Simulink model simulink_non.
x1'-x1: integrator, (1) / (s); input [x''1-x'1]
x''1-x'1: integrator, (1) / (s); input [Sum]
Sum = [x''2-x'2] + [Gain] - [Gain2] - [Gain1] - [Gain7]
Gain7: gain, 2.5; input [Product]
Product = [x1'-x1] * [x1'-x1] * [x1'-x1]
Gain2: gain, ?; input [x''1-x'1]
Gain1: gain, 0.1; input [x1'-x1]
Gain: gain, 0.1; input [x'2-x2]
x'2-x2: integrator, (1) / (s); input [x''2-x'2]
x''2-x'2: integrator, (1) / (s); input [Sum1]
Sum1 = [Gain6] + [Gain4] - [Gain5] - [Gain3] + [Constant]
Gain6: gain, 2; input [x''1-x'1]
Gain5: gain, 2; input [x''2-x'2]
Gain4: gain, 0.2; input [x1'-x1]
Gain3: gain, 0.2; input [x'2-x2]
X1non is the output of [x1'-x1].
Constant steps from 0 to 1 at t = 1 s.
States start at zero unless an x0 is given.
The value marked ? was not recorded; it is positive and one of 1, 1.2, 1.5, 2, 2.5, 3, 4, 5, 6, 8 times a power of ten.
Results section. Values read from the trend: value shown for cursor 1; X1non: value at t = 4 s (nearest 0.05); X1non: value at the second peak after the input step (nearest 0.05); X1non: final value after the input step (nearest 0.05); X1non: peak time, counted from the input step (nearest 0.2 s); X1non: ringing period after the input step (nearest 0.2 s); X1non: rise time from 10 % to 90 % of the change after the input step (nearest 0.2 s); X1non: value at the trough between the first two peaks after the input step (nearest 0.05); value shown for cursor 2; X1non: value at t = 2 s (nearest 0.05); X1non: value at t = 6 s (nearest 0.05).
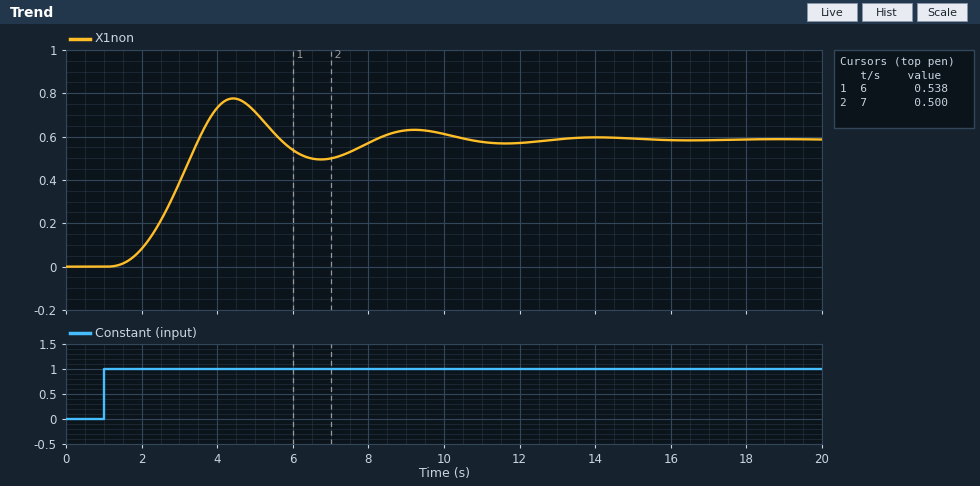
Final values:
0.538
0.75
0.65
0.60
3.4 s
4.8 s
1.4 s
0.50
0.500
0.10
0.55
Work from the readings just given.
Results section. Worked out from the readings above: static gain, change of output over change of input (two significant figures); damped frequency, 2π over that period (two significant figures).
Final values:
0.60
1.3 rad/s
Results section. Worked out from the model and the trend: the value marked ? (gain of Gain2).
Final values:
1.5
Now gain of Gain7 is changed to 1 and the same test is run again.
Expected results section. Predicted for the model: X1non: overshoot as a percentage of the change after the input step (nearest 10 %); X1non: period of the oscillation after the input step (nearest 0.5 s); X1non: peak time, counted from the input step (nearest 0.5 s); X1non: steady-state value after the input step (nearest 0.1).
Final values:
30 %
5.5 s
4.0 s
0.8
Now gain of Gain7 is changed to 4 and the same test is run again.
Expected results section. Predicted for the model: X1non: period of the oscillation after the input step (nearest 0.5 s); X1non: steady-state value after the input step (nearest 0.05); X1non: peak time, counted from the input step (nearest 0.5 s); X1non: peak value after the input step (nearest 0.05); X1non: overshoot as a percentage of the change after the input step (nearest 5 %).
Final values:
4.5 s
0.50
3.0 s
0.65
35 %
